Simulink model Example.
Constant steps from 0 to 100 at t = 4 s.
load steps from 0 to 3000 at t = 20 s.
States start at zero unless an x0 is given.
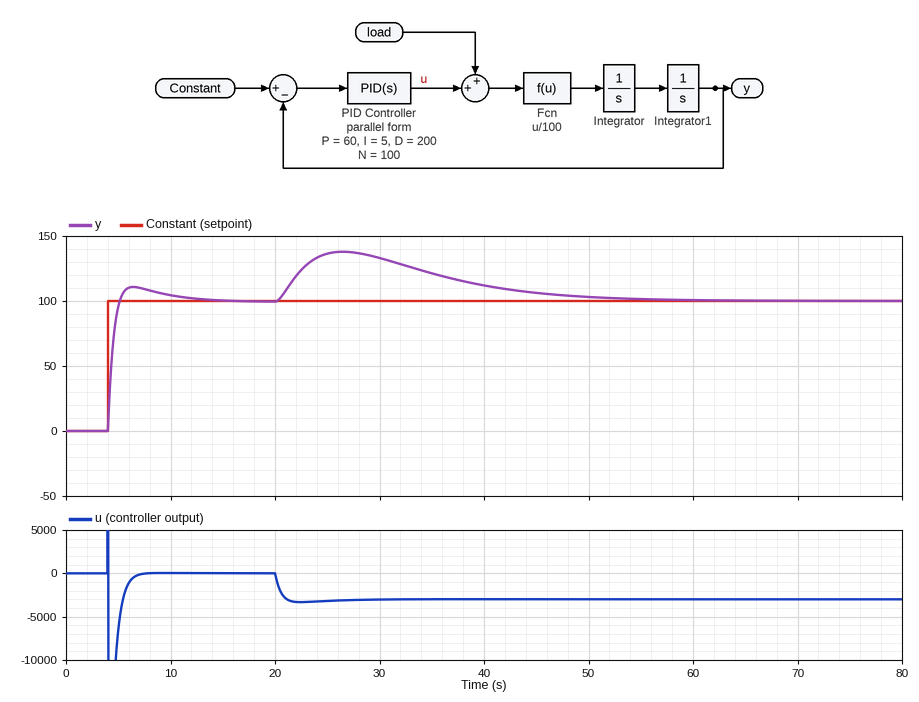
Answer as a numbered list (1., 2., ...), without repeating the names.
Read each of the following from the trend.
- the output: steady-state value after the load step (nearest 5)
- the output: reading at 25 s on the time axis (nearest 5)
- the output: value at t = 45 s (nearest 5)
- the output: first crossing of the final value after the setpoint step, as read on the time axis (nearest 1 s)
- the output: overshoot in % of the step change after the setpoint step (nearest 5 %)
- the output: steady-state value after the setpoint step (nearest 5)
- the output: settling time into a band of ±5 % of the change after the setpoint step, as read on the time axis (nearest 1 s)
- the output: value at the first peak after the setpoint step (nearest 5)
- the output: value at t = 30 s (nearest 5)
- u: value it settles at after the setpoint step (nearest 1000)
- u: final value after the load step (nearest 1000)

1. 100
2. 135
3. 105
4. 5 s
5. 10 %
6. 100
7. 10 s
8. 110
9. 135
10. 0
11. -3000
